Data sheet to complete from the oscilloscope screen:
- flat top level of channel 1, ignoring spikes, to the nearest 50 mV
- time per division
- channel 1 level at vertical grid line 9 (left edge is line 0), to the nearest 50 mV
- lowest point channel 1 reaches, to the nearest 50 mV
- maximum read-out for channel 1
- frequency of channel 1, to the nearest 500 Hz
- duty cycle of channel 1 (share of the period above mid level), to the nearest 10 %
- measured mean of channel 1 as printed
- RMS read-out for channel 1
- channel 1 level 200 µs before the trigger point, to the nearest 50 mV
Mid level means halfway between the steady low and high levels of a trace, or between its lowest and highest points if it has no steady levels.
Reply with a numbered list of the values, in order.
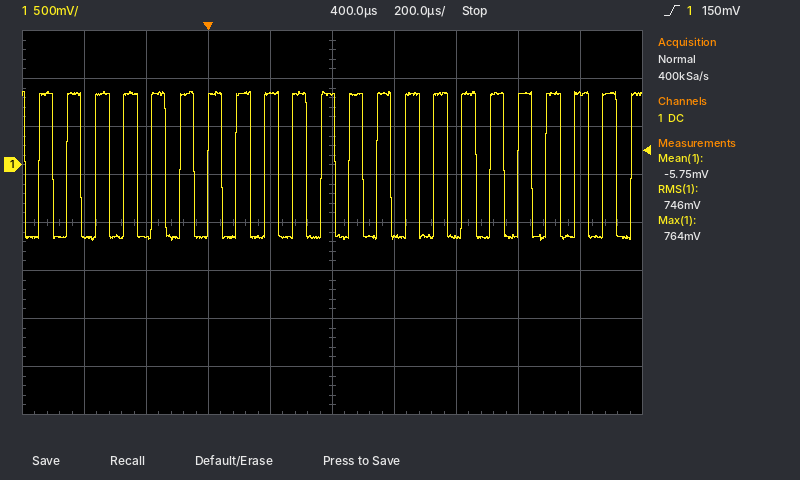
1. 750 mV
2. 200 µs
3. 750 mV
4. -800 mV
5. 764 mV
6. 11.0 kHz
7. 50 %
8. -5.75 mV
9. 746 mV
10. -750 mV
